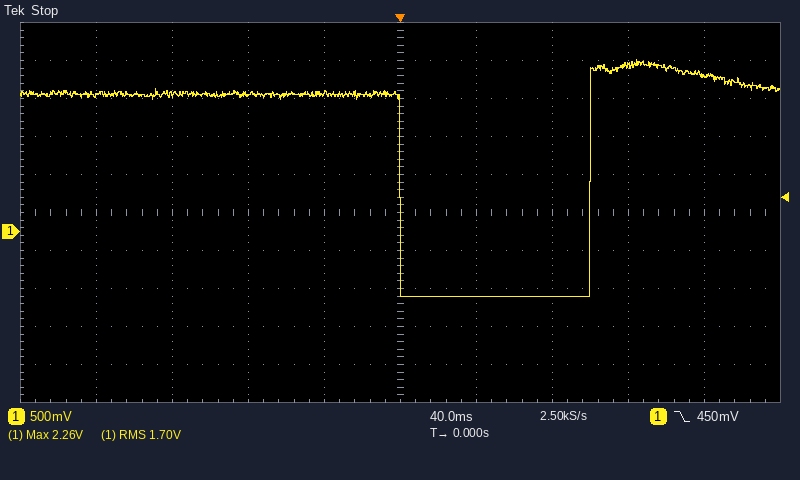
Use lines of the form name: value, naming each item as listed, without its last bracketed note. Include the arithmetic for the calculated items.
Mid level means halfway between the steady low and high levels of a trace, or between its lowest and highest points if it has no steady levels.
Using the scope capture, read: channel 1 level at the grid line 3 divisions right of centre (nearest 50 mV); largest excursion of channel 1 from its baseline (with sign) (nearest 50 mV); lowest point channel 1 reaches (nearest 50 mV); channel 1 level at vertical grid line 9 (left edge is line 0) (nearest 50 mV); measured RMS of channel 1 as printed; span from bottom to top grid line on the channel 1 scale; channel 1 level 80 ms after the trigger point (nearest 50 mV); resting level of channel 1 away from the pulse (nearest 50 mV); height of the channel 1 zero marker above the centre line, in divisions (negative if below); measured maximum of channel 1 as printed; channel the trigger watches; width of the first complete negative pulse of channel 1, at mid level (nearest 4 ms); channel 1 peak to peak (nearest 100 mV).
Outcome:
channel 1 level at the grid line 3 divisions right of centre: 2.20 V
largest excursion of channel 1 from its baseline (with sign): -850 mV − (1.80 V) = -2.65 V
lowest point channel 1 reaches: -850 mV
channel 1 level at vertical grid line 9 (left edge is line 0): 2.05 V
measured RMS of channel 1 as printed: 1.70 V
span from bottom to top grid line on the channel 1 scale: 5 V
channel 1 level 80 ms after the trigger point: -850 mV
resting level of channel 1 away from the pulse: 1.80 V
height of the channel 1 zero marker above the centre line, in divisions: -0.5 div
measured maximum of channel 1 as printed: 2.26 V
channel the trigger watches: channel 1
width of the first complete negative pulse of channel 1, at mid level: 100 ms
channel 1 peak to peak: 3.10 V
